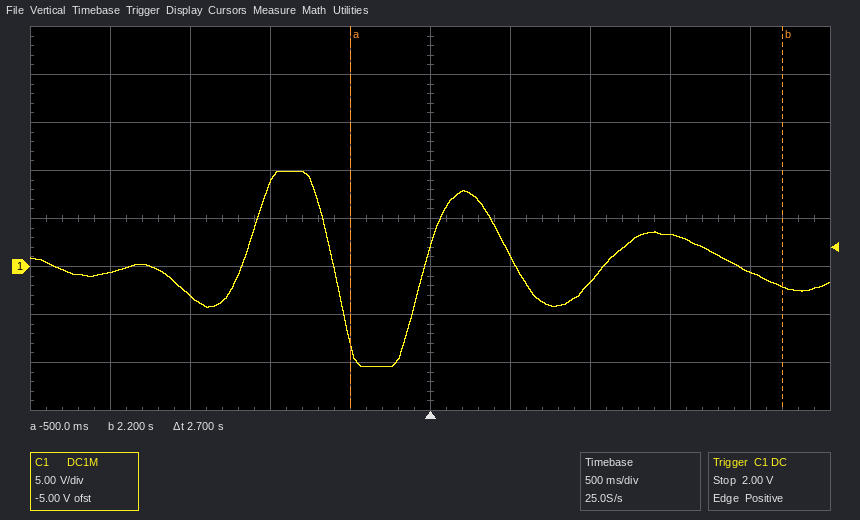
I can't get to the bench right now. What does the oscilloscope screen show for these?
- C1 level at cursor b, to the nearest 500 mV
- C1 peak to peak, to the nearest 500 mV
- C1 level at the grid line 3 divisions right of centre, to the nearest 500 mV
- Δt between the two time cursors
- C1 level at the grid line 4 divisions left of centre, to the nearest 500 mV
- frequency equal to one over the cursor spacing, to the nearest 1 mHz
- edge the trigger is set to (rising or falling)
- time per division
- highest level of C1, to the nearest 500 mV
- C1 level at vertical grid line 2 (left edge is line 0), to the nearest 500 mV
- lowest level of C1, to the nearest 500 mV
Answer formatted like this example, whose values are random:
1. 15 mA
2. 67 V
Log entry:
1. -2.0 V
2. 20.5 V
3. 3.5 V
4. 2.7 s
5. -500 mV
6. 370 mHz
7. rising
8. 500 ms
9. 10.0 V
10. -3.0 V
11. -10.5 V
